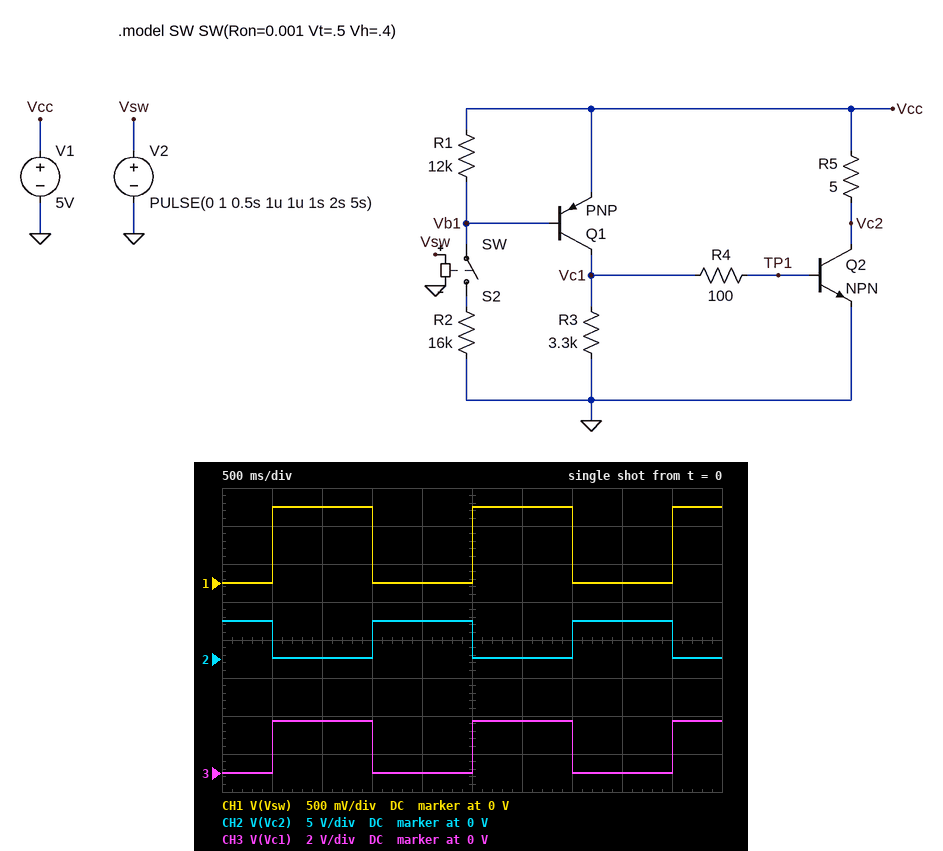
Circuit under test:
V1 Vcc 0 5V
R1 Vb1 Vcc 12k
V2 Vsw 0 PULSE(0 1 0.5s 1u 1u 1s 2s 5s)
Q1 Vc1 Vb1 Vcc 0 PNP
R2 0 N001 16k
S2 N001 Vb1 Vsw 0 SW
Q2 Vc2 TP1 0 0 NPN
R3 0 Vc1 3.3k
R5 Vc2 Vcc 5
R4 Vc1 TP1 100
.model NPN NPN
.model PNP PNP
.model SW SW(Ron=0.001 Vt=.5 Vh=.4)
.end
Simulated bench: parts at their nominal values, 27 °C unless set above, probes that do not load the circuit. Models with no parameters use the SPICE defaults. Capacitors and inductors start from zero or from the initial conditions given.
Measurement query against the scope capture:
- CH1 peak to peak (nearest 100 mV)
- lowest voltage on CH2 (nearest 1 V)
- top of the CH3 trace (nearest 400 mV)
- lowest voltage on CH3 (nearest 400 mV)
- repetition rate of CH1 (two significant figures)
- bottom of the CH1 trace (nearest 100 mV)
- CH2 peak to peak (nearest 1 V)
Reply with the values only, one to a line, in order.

1.0 V
0 V
2.8 V
0 V
500 mHz
0 V
5 V
